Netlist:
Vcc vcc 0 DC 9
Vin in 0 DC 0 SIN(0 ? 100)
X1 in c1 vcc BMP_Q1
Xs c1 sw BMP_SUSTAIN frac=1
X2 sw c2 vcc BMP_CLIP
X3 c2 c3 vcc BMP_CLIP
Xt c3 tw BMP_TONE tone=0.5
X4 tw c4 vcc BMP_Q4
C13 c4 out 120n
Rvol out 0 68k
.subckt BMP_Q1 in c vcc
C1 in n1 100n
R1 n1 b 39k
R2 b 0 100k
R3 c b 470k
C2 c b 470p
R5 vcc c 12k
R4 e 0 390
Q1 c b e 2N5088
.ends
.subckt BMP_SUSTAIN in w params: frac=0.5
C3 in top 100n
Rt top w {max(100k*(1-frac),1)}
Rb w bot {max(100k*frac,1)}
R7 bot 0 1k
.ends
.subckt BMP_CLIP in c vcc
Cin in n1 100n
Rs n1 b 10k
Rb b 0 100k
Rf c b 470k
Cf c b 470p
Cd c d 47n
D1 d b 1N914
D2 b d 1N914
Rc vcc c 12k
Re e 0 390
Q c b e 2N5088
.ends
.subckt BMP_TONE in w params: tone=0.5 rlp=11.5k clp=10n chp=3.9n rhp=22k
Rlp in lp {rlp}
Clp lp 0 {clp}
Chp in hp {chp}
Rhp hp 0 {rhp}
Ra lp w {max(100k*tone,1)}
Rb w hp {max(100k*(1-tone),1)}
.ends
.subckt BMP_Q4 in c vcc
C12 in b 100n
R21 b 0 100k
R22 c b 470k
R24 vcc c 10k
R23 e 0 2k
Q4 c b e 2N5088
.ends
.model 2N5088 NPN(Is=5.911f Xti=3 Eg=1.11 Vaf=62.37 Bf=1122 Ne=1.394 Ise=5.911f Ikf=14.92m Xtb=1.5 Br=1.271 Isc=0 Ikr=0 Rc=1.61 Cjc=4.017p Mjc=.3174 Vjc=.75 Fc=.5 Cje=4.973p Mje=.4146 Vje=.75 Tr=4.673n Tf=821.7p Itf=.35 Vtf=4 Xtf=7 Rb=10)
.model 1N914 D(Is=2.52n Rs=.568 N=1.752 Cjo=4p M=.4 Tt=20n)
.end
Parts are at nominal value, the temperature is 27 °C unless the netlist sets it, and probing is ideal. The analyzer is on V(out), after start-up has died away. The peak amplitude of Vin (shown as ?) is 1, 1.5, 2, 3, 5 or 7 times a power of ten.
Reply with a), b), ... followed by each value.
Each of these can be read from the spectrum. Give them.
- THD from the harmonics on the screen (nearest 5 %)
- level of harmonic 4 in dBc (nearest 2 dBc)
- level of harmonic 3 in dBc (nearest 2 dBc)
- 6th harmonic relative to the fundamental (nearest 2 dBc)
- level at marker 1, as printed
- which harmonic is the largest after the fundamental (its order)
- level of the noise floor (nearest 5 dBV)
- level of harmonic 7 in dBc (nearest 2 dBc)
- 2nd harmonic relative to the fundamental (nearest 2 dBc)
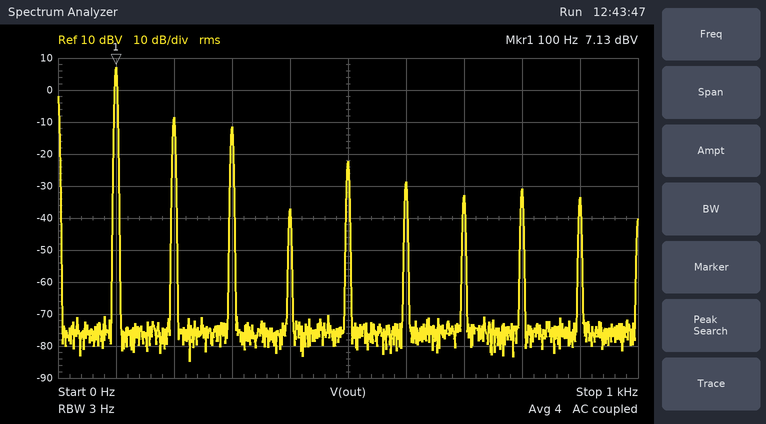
a) 20 %
b) -44 dBc
c) -18 dBc
d) -36 dBc
e) 7.13 dBV
f) 2
g) -75 dBV
h) -40 dBc
i) -16 dBc
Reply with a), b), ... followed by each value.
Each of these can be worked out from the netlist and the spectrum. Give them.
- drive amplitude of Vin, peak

a) 500 mV
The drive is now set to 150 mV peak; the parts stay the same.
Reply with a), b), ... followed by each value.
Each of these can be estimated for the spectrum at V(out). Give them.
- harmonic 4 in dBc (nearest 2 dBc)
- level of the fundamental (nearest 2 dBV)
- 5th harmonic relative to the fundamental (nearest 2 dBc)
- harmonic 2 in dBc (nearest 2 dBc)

a) -40 dBc
b) 2 dBV
c) -24 dBc
d) -34 dBc
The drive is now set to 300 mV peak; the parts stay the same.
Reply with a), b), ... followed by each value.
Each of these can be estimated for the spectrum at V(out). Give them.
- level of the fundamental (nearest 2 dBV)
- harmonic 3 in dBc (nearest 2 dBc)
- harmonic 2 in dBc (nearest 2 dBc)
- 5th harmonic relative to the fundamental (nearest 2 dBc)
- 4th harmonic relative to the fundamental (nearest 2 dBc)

a) 6 dBV
b) -28 dBc
c) -18 dBc
d) -36 dBc
e) -24 dBc
